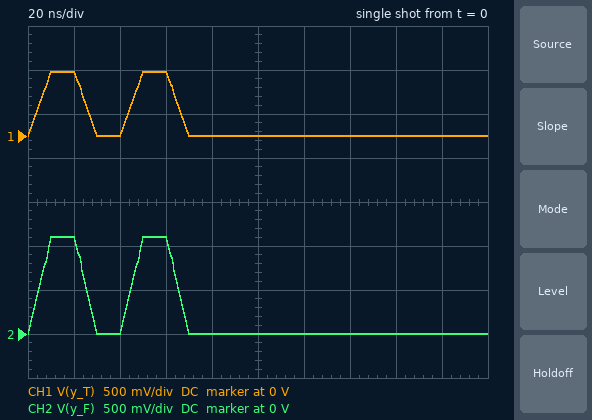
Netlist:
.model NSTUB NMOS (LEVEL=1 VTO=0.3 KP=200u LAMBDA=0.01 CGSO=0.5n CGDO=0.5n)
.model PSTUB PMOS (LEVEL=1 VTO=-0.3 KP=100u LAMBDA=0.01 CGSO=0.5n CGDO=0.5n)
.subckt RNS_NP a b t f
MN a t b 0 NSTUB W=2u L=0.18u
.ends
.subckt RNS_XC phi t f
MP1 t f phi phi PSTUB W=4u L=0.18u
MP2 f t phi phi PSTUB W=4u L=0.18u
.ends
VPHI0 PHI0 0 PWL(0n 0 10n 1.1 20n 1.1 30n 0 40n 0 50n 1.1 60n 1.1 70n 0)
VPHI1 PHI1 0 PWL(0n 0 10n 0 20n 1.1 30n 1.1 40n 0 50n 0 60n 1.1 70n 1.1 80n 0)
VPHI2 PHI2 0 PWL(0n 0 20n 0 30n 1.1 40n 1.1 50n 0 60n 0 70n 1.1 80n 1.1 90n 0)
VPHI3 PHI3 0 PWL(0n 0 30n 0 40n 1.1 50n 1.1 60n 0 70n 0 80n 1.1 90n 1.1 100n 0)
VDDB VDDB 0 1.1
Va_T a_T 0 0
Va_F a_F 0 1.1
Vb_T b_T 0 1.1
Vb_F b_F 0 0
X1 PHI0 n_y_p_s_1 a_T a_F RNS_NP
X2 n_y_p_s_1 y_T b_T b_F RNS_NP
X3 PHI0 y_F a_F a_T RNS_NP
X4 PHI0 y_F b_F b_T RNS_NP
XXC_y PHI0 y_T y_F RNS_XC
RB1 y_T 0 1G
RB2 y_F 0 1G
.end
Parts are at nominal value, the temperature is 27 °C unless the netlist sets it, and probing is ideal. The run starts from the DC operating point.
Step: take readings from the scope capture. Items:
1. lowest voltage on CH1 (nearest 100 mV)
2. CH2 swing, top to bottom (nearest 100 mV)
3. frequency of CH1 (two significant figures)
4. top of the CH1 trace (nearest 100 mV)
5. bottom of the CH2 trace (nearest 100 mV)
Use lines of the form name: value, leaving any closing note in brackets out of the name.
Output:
lowest voltage on CH1: 0 V
CH2 swing, top to bottom: 1.1 V
frequency of CH1: 25 MHz
top of the CH1 trace: 700 mV
bottom of the CH2 trace: 0 V
